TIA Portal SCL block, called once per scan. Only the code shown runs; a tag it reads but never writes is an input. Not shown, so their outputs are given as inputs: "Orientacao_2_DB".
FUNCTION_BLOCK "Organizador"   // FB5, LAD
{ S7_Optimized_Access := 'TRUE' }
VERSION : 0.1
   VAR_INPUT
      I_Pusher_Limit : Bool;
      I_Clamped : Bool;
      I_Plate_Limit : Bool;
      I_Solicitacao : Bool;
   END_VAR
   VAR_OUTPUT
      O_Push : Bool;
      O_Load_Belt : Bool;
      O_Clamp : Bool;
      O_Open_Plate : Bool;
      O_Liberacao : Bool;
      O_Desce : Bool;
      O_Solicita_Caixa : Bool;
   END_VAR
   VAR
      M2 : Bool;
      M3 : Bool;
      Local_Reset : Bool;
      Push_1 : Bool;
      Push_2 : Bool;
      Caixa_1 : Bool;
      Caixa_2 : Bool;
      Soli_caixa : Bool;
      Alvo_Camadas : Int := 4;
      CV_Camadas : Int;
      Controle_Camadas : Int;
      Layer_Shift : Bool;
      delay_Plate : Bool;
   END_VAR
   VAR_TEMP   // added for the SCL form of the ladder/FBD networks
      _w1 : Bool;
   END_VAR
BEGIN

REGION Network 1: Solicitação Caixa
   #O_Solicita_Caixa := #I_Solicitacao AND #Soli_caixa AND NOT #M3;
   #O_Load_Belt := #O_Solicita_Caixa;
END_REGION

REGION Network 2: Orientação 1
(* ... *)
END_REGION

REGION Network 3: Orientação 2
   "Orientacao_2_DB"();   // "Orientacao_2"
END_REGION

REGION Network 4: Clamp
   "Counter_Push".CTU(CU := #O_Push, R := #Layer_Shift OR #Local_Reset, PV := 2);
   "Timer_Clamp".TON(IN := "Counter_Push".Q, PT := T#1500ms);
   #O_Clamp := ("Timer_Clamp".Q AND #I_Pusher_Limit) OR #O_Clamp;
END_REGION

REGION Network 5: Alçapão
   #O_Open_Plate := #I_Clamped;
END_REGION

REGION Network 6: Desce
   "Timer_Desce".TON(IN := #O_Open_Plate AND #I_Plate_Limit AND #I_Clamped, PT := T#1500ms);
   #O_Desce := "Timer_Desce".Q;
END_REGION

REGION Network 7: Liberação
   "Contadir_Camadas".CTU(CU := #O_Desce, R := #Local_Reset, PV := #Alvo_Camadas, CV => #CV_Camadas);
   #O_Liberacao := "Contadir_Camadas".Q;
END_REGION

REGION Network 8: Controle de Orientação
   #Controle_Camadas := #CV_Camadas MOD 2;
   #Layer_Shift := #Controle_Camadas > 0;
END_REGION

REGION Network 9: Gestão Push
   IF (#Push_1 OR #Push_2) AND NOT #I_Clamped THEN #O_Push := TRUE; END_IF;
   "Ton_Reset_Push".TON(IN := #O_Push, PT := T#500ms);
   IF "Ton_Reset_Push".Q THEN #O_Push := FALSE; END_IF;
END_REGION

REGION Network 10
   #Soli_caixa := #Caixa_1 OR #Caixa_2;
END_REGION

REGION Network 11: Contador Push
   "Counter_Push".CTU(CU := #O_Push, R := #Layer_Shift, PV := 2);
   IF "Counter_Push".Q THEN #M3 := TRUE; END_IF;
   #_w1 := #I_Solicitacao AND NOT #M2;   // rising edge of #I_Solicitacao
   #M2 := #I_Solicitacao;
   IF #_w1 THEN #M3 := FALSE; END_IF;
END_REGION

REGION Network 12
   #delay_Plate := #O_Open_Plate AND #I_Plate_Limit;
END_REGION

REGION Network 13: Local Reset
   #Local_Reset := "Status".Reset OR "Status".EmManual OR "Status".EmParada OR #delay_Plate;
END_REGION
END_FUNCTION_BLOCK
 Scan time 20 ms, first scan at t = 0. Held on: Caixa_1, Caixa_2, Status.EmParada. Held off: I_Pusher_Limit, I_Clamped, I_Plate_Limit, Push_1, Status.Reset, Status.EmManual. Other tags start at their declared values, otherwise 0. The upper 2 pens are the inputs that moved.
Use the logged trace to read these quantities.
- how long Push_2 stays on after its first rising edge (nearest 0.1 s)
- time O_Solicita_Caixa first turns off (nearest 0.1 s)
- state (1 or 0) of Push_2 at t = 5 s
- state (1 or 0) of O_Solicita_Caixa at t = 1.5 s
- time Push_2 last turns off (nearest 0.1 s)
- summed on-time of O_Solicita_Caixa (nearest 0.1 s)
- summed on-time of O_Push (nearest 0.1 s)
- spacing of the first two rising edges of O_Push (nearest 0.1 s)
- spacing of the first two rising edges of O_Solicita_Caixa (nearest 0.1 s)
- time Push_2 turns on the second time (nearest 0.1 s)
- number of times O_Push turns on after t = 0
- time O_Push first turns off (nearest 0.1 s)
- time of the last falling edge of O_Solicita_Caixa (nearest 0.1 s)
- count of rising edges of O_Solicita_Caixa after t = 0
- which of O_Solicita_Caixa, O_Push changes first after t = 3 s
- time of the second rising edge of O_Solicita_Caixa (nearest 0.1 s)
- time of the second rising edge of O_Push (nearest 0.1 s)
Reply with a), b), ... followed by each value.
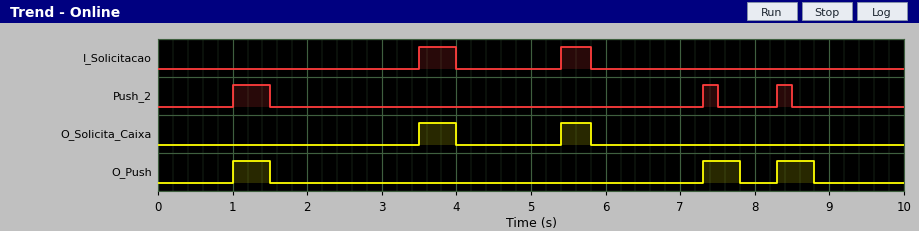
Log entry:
a) 0.5 s
b) 4.0 s
c) 0
d) 0
e) 8.5 s
f) 0.9 s
g) 1.5 s
h) 6.3 s
i) 1.9 s
j) 7.3 s
k) 3
l) 1.5 s
m) 5.8 s
n) 2
o) O_Solicita_Caixa
p) 5.4 s
q) 7.3 s
